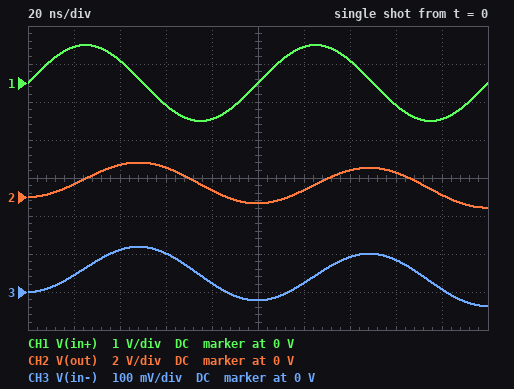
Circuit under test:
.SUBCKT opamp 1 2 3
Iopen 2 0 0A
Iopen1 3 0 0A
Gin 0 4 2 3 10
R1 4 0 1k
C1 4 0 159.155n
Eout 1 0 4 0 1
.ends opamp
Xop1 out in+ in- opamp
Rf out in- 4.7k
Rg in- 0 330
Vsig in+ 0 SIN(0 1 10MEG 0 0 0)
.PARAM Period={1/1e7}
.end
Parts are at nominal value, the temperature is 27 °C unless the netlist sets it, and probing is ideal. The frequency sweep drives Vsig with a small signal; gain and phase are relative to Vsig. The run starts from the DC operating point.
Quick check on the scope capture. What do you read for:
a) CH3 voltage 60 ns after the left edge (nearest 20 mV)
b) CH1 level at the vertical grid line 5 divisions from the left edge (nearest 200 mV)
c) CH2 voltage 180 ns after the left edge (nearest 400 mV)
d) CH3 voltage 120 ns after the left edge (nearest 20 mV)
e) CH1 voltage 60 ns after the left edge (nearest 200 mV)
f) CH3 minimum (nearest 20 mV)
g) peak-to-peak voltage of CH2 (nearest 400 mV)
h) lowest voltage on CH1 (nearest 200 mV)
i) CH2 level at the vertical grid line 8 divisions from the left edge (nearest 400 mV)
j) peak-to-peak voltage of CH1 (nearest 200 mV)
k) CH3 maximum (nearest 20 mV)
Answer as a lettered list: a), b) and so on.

a) 100 mV
b) 0 V
c) 0 V
d) 20 mV
e) -600 mV
f) -40 mV
g) 2.4 V
h) -1.0 V
i) 1.2 V
j) 2.0 V
k) 120 mV
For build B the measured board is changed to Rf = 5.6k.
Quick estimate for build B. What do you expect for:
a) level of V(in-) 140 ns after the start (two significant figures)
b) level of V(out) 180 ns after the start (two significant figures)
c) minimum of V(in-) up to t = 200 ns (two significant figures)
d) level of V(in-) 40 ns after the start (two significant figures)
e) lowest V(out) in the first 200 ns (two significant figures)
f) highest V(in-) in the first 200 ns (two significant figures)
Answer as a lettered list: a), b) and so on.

a) 81 mV
b) 170 mV
c) -28 mV
d) 95 mV
e) -500 mV
f) 100 mV
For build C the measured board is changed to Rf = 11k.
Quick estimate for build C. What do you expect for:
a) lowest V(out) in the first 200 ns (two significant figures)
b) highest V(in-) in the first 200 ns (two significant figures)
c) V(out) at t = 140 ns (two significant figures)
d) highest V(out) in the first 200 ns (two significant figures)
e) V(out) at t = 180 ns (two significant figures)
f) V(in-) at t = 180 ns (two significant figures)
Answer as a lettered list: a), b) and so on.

a) -310 mV
b) 56 mV
c) 1.6 V
d) 1.9 V
e) 380 mV
f) 11 mV
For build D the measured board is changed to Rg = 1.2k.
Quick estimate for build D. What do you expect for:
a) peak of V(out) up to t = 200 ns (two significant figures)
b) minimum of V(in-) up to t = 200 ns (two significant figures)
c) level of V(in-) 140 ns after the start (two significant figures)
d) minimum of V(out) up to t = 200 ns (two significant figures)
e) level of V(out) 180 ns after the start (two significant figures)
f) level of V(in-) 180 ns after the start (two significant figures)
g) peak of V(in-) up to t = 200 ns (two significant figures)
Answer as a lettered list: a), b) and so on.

a) 1.5 V
b) -180 mV
c) 210 mV
d) -900 mV
e) -390 mV
f) -79 mV
g) 310 mV
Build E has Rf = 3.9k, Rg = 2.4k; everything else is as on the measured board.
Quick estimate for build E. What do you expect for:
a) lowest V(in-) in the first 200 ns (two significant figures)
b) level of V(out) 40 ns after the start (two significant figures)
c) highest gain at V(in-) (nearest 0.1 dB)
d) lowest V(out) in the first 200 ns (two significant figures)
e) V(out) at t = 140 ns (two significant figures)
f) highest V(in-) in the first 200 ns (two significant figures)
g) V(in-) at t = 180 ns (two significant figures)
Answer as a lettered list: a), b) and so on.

a) -350 mV
b) 1.2 V
c) 0 dB
d) -930 mV
e) 930 mV
f) 470 mV
g) -220 mV
